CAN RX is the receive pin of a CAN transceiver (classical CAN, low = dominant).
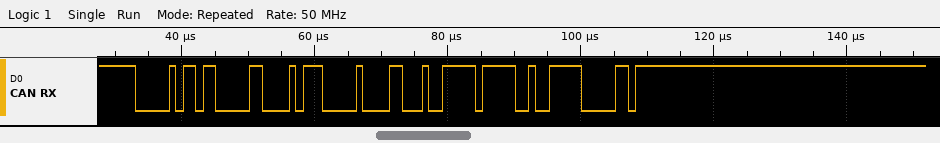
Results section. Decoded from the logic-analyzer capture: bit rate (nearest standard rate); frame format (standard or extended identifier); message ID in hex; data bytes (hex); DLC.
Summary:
1000 kbit/s
standard
0x036
2E 00 C4 FF
4
